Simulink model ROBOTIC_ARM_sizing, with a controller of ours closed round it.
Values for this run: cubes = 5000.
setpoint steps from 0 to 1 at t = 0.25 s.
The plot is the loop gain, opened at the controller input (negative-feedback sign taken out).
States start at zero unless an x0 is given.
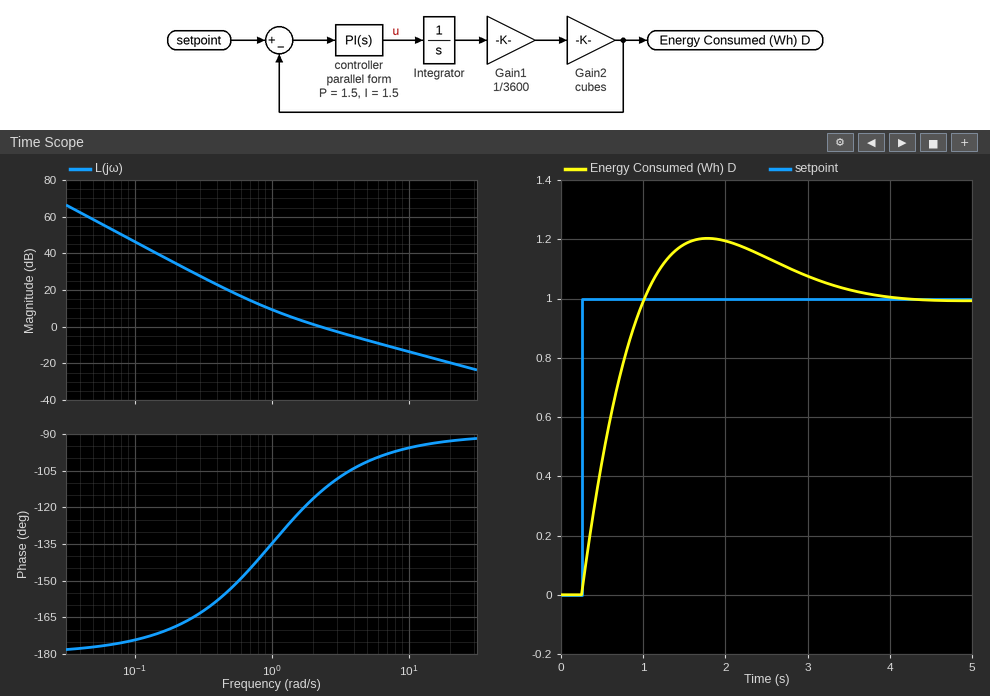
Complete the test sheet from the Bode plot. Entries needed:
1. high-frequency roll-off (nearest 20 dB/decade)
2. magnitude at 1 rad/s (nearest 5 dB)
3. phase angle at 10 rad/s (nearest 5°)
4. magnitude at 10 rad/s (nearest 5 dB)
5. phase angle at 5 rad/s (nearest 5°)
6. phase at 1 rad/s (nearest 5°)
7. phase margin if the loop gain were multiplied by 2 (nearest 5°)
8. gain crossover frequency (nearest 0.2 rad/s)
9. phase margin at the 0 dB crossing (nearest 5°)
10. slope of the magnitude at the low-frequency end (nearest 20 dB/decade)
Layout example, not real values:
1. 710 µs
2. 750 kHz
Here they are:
1. -20 dB/decade
2. 10 dB
3. -95°
4. -15 dB
5. -100°
6. -135°
7. 75°
8. 2.2 rad/s
9. 65°
10. -40 dB/decade
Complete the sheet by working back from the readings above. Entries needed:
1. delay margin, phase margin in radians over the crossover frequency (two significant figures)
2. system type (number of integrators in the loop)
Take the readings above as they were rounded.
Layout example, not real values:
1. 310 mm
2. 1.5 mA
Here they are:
1. 0.52 s
2. 2
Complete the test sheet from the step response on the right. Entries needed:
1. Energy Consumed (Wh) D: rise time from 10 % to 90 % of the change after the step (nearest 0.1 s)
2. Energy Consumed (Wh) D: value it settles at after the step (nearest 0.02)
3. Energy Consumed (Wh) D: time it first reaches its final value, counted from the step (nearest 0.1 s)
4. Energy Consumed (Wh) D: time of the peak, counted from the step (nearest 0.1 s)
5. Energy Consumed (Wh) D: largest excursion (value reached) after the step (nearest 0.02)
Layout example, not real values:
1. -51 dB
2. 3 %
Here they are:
1. 0.6 s
2. 1.00
3. 0.8 s
4. 1.5 s
5. 1.20
